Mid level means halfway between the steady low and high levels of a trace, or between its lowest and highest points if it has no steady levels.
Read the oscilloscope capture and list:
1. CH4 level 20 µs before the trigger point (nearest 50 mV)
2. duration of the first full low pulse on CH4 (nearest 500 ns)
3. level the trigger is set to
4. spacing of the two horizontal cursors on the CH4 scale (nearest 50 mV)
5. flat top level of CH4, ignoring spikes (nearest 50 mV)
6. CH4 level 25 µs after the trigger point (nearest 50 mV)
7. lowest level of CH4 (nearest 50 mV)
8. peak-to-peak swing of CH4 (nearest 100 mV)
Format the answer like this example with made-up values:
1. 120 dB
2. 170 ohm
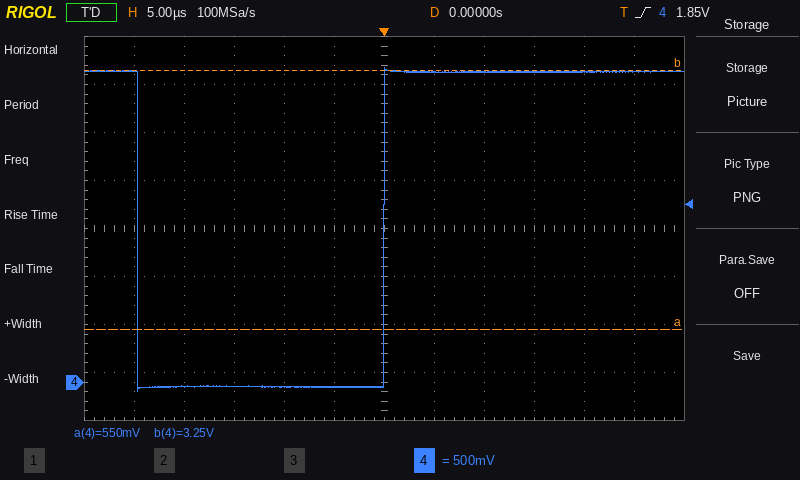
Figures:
1. -50 mV
2. 24.5 µs
3. 1.85 V
4. 2.70 V
5. 3.25 V
6. 3.25 V
7. -100 mV
8. 3.40 V
